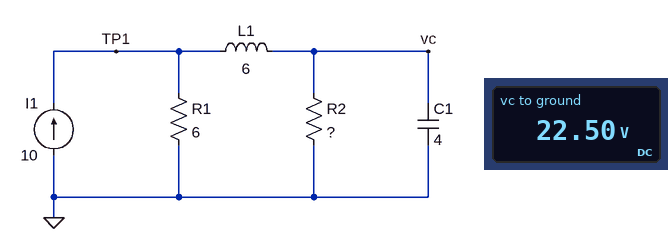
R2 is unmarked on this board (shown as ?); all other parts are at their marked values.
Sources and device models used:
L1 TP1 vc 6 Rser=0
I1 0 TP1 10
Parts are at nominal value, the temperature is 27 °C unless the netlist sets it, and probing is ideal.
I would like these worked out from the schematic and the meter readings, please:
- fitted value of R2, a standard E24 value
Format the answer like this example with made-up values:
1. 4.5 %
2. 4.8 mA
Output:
1. 3.6 Ω
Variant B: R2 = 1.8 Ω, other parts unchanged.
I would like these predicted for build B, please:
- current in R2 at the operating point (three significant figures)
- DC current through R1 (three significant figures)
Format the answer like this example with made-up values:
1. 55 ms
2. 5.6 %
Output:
1. 7.69 A
2. 2.31 A
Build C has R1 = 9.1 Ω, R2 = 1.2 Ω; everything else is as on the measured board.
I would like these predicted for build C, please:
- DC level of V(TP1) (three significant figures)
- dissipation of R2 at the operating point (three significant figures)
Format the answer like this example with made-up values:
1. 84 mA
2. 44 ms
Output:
1. 10.6 V
2. 93.7 W
